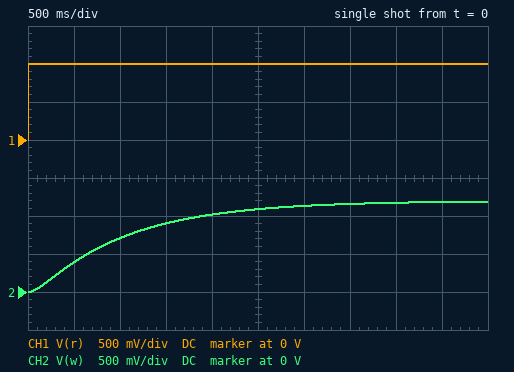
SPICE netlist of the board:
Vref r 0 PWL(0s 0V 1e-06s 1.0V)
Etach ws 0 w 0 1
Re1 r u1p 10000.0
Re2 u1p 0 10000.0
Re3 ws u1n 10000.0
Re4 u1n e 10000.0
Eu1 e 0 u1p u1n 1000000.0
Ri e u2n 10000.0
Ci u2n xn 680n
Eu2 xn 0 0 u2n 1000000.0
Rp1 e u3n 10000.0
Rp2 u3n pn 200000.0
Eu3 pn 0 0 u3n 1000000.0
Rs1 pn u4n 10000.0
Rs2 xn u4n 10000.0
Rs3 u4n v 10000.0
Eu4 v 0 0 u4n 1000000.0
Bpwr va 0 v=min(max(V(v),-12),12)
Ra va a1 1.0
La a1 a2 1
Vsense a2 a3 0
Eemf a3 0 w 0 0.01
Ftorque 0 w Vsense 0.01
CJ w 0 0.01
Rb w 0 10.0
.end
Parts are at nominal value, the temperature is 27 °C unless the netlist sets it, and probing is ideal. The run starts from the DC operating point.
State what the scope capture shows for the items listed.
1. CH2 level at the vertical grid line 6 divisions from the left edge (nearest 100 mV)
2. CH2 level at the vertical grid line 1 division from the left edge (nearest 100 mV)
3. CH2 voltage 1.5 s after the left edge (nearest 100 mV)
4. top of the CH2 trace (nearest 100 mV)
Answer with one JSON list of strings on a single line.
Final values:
["1.1 V", "400 mV", "900 mV", "1.2 V"]
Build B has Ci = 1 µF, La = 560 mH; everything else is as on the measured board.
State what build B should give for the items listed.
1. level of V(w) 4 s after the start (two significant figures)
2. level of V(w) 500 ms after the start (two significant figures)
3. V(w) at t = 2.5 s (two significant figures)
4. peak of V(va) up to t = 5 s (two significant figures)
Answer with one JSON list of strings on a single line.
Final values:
["960 mV", "600 mV", "1.2 V", "12 V"]
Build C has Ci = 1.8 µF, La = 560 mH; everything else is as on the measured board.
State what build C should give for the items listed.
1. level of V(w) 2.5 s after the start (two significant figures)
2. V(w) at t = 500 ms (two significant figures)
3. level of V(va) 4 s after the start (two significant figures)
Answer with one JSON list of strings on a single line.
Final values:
["1.2 V", "600 mV", "10 V"]
